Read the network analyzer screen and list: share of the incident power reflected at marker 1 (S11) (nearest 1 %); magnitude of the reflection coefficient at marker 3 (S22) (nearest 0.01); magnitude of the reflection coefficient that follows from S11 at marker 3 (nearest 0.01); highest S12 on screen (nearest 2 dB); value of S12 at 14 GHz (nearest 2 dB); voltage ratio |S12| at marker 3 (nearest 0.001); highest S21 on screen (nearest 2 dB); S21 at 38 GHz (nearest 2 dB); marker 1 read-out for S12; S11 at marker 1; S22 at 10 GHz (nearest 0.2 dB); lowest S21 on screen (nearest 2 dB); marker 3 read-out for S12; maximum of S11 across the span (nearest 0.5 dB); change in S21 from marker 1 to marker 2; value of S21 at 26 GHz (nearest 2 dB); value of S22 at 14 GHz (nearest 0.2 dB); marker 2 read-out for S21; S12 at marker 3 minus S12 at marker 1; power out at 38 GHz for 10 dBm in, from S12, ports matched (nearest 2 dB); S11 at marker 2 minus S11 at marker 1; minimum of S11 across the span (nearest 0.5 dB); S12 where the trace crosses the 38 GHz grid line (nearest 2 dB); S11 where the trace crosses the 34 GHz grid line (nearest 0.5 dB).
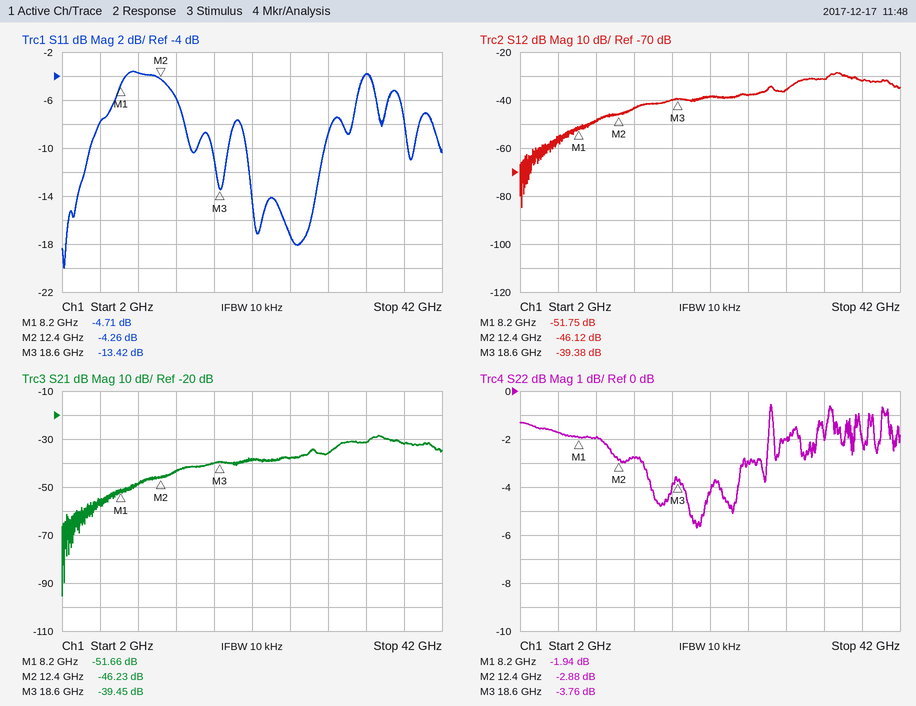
34 %
0.65
0.21
-28 dB
-44 dB
0.011
-28 dB
-32 dB
-51.75 dB
-4.71 dB
-2.0 dB
-96 dB
-39.38 dB
-3.5 dB
5.43 dB
-38 dB
-2.8 dB
-46.23 dB
12.37 dB
-22 dBm
0.45 dB
-20.0 dB
-32 dB
-4.0 dB
